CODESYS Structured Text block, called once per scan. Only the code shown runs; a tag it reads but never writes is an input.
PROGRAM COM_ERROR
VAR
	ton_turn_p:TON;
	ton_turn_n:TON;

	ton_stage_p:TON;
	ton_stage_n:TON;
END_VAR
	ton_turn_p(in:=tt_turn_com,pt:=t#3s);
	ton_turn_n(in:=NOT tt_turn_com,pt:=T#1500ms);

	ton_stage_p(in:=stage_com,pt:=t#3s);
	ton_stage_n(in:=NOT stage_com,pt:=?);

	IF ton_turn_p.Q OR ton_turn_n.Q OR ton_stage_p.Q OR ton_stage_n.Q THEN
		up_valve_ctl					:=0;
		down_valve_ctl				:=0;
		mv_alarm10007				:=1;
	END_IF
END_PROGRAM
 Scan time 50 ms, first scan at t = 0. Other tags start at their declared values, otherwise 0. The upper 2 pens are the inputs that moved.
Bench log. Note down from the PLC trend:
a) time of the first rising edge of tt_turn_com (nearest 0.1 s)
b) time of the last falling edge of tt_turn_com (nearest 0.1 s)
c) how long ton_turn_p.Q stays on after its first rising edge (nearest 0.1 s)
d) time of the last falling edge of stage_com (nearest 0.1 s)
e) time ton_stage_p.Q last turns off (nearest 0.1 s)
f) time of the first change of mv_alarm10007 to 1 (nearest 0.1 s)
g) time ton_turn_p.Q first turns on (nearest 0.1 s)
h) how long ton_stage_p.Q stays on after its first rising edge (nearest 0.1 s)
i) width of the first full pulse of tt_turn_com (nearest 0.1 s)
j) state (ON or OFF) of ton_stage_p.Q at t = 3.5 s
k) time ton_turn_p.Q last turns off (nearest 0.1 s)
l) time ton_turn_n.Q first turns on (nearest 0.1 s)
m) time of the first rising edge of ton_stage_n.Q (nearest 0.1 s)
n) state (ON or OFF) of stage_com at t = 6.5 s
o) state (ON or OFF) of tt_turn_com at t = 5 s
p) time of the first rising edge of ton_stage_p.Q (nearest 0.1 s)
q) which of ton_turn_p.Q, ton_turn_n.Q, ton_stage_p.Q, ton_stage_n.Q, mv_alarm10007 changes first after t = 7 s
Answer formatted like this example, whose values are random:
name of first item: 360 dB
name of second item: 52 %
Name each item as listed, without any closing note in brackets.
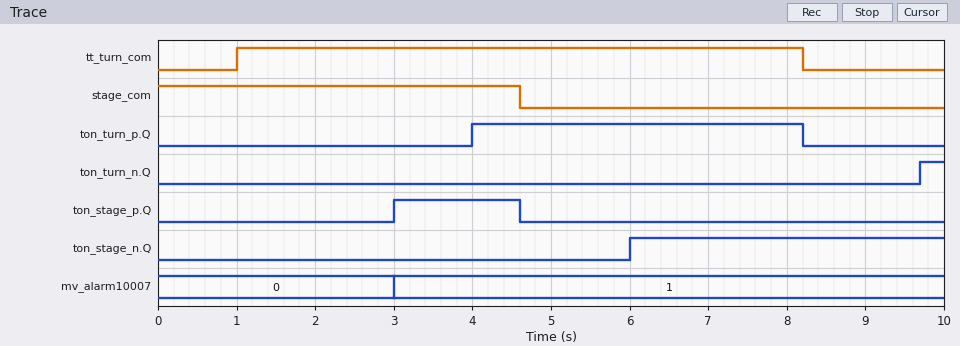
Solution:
time of the first rising edge of tt_turn_com: 1.0 s
time of the last falling edge of tt_turn_com: 8.2 s
how long ton_turn_p.Q stays on after its first rising edge: 4.2 s
time of the last falling edge of stage_com: 4.6 s
time ton_stage_p.Q last turns off: 4.6 s
time of the first change of mv_alarm10007 to 1: 3.0 s
time ton_turn_p.Q first turns on: 4.0 s
how long ton_stage_p.Q stays on after its first rising edge: 1.6 s
width of the first full pulse of tt_turn_com: 7.2 s
state (ON or OFF) of ton_stage_p.Q at t = 3.5 s: ON
time ton_turn_p.Q last turns off: 8.2 s
time ton_turn_n.Q first turns on: 9.7 s
time of the first rising edge of ton_stage_n.Q: 6.0 s
state (ON or OFF) of stage_com at t = 6.5 s: OFF
state (ON or OFF) of tt_turn_com at t = 5 s: ON
time of the first rising edge of ton_stage_p.Q: 3.0 s
which of ton_turn_p.Q, ton_turn_n.Q, ton_stage_p.Q, ton_stage_n.Q, mv_alarm10007 changes first after t = 7 s: ton_turn_p.Q
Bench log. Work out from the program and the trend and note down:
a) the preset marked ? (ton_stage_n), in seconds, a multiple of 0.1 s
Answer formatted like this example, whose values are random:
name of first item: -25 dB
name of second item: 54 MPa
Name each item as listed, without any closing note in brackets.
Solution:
the preset marked ? (ton_stage_n), in seconds, a multiple of 0.1 s: 1.4 s
